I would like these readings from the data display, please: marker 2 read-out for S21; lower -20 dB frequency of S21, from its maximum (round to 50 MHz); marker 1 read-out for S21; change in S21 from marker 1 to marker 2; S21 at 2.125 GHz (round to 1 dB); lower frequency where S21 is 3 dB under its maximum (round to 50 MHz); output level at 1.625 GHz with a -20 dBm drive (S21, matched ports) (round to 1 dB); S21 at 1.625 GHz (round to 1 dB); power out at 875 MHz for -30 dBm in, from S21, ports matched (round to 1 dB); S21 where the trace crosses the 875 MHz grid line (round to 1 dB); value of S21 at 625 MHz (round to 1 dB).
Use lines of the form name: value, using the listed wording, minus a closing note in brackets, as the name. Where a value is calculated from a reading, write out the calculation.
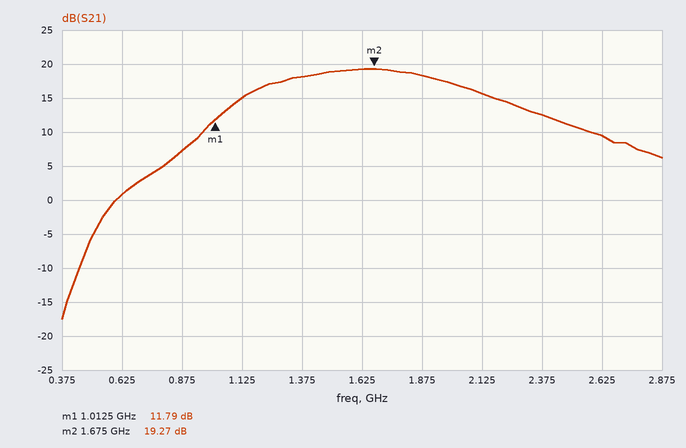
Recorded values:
marker 2 read-out for S21: 19.27 dB
lower -20 dB frequency of S21, from its maximum: 600 MHz
marker 1 read-out for S21: 11.79 dB
change in S21 from marker 1 to marker 2: 19.27 − (11.79) = 7.48 dB
S21 at 2.125 GHz: 16 dB
lower frequency where S21 is 3 dB under its maximum: 1.20 GHz
output level at 1.625 GHz with a -20 dBm drive (S21, matched ports): -20 dBm + (19 dB) = -1 dBm
S21 at 1.625 GHz: 19 dB
power out at 875 MHz for -30 dBm in, from S21, ports matched: -30 dBm + (7 dB) = -23 dBm
S21 where the trace crosses the 875 MHz grid line: 7 dB
value of S21 at 625 MHz: 1 dB
